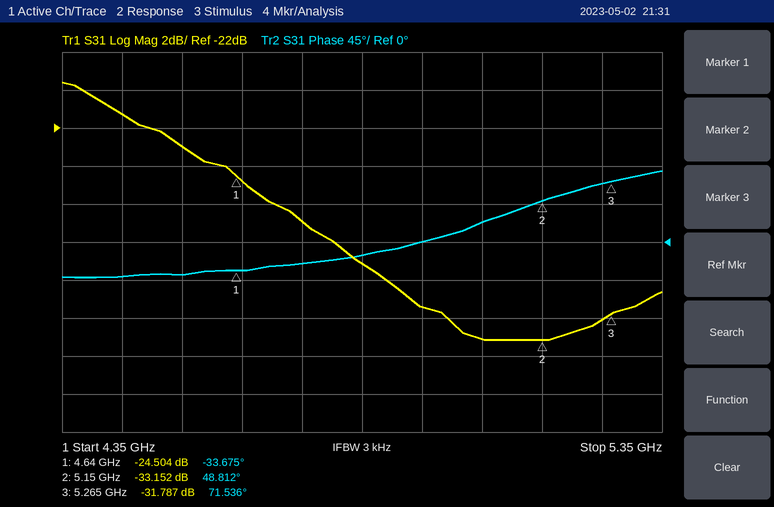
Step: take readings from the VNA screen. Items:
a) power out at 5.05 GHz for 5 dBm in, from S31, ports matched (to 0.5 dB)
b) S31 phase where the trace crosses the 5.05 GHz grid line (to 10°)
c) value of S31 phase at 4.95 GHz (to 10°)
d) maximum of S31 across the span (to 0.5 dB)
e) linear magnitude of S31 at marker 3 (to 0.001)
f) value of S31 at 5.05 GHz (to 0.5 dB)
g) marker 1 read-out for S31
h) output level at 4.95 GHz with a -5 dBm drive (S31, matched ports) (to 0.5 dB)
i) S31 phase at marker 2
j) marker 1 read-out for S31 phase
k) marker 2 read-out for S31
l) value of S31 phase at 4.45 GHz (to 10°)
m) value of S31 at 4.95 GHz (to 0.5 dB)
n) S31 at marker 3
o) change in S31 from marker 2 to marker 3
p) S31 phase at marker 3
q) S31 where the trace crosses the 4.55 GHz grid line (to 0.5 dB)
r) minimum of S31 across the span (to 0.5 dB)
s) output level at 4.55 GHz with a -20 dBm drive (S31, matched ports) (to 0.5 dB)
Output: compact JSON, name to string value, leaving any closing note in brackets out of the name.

{"power out at 5.05 GHz for 5 dBm in, from S31, ports matched": "-28.0 dBm", "S31 phase where the trace crosses the 5.05 GHz grid line": "20°", "value of S31 phase at 4.95 GHz": "0°", "maximum of S31 across the span": "-19.5 dB", "linear magnitude of S31 at marker 3": "0.026", "value of S31 at 5.05 GHz": "-33.0 dB", "marker 1 read-out for S31": "-24.504 dB", "output level at 4.95 GHz with a -5 dBm drive (S31, matched ports)": "-36.5 dBm", "S31 phase at marker 2": "48.812°", "marker 1 read-out for S31 phase": "-33.675°", "marker 2 read-out for S31": "-33.152 dB", "value of S31 phase at 4.45 GHz": "-40°", "value of S31 at 4.95 GHz": "-31.5 dB", "S31 at marker 3": "-31.787 dB", "change in S31 from marker 2 to marker 3": "1.365 dB", "S31 phase at marker 3": "71.536°", "S31 where the trace crosses the 4.55 GHz grid line": "-23.0 dB", "minimum of S31 across the span": "-33.0 dB", "output level at 4.55 GHz with a -20 dBm drive (S31, matched ports)": "-43.0 dBm"}
